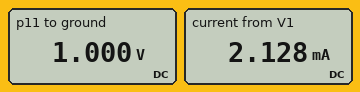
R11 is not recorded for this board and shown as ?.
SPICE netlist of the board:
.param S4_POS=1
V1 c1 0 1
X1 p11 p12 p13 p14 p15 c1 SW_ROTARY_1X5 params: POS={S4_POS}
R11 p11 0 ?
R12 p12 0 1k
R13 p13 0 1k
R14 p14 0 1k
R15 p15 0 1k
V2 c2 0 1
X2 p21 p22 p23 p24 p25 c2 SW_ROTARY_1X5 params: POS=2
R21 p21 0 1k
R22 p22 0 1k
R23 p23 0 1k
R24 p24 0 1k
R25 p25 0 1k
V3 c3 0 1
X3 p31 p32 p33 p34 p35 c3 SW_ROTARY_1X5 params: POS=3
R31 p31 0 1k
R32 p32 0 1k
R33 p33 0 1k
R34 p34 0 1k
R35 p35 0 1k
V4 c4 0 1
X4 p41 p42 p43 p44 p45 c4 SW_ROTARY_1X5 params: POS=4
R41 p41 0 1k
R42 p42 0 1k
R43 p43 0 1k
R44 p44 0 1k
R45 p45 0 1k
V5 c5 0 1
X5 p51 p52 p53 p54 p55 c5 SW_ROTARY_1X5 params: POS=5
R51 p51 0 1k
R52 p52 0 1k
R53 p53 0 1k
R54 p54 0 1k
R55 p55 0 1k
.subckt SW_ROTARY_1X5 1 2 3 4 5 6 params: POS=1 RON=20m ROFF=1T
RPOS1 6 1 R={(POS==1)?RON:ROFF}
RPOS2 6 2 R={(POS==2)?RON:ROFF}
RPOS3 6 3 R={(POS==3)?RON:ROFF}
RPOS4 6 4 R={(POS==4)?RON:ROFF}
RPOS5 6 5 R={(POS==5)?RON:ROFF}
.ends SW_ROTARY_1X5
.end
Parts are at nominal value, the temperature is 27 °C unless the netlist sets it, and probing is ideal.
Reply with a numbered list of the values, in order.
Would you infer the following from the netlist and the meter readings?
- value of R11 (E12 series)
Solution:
1. 470 Ω
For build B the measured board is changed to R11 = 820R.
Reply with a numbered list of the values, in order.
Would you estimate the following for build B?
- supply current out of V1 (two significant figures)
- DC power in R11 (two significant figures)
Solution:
1. 1.2 mA
2. 1.2 mW
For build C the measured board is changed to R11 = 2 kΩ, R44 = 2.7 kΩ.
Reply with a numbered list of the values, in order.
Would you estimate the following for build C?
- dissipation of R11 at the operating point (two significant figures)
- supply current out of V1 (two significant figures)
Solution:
1. 500 µW
2. 500 µA
